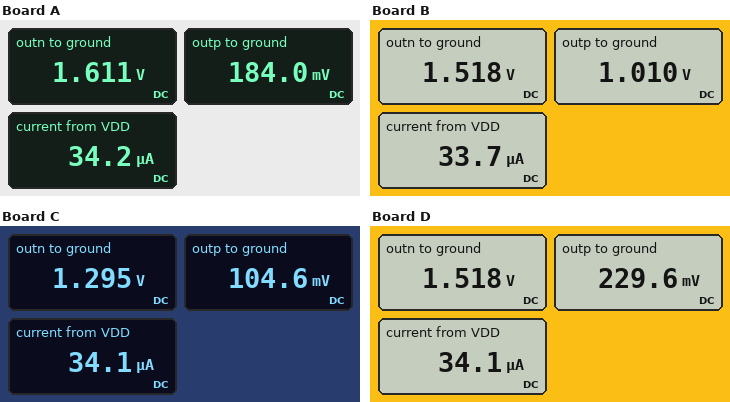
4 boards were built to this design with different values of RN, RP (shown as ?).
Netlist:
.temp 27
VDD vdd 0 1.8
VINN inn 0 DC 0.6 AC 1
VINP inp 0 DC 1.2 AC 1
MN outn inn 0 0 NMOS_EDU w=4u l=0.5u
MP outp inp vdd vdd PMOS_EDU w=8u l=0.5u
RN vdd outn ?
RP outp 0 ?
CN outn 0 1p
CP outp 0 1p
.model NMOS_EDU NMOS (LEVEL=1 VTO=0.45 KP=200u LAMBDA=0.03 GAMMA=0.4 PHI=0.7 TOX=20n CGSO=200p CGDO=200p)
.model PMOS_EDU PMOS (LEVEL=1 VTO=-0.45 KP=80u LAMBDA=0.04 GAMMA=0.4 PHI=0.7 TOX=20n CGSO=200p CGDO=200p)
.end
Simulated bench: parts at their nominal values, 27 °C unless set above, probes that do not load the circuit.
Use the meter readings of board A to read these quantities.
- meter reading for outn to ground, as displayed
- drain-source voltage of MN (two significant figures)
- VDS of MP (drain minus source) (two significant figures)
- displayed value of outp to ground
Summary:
1.611 V
1.6 V
-1.6 V
184.0 mV
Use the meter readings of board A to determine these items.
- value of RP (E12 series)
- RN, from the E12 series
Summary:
12 kΩ
10 kΩ
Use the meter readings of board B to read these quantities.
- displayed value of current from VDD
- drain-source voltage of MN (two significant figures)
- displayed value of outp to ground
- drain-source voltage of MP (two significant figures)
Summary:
33.7 µA
1.5 V
1.010 V
-790 mV
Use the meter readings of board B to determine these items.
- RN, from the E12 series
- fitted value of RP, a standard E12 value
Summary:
15 kΩ
68 kΩ
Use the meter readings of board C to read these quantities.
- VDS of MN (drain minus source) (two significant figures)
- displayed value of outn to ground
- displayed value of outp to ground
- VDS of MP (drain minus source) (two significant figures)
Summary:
1.3 V
1.295 V
104.6 mV
-1.7 V
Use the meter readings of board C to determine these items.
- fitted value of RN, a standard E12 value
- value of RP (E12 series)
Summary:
27 kΩ
6.8 kΩ
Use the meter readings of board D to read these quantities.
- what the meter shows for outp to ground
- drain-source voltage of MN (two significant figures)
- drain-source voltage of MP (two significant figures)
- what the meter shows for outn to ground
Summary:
229.6 mV
1.5 V
-1.6 V
1.518 V
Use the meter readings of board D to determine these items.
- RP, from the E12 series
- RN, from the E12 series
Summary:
15 kΩ
15 kΩ
